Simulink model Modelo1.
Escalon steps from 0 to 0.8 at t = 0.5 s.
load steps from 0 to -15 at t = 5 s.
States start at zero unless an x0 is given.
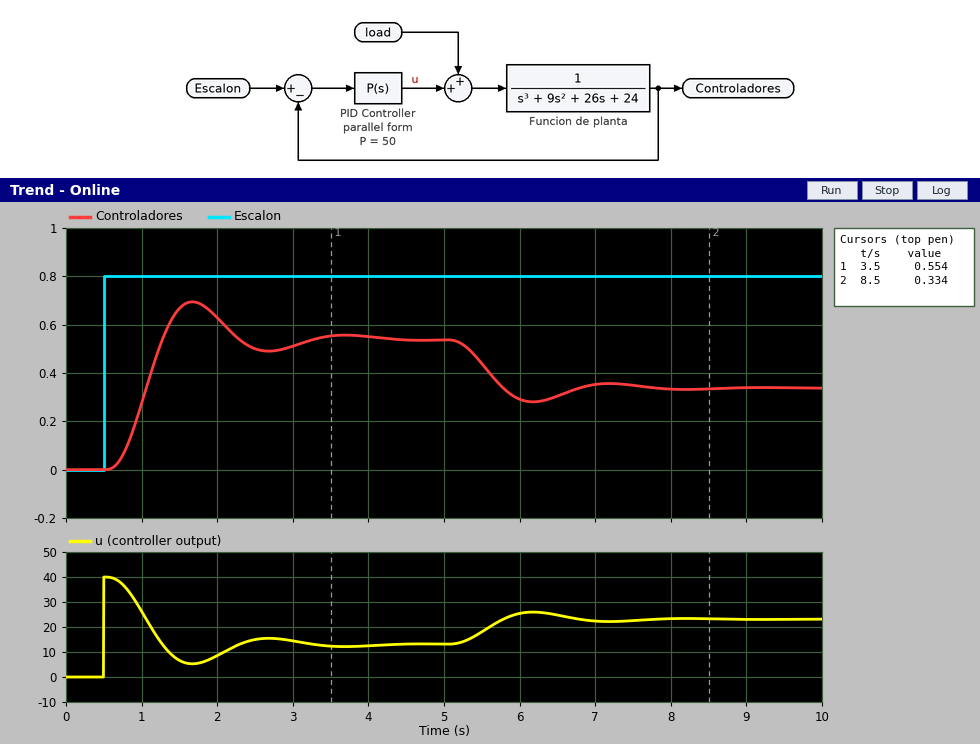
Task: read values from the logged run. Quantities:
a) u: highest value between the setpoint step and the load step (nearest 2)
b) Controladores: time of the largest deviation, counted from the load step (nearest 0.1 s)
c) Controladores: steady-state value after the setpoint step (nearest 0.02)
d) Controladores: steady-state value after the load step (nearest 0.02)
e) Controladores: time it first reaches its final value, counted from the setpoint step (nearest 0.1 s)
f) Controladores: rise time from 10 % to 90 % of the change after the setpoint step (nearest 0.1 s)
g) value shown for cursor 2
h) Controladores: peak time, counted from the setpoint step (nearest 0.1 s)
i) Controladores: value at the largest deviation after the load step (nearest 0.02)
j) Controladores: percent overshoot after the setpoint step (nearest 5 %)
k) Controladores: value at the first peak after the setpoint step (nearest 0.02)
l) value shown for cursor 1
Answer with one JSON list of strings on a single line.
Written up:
["40", "1.2 s", "0.54", "0.34", "0.8 s", "0.5 s", "0.334", "1.2 s", "0.28", "30 %", "0.70", "0.554"]
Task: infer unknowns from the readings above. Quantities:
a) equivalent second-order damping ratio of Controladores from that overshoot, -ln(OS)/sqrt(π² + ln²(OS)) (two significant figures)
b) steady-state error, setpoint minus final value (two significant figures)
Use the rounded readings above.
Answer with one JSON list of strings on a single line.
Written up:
["0.36", "0.26"]
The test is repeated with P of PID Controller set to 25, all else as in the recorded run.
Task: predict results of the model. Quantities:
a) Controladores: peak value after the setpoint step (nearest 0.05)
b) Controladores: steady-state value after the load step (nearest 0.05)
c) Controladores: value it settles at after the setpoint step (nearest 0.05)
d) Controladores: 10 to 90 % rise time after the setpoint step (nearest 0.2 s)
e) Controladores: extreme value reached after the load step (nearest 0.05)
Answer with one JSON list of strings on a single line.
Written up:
["0.45", "0.10", "0.40", "0.6 s", "0.05"]
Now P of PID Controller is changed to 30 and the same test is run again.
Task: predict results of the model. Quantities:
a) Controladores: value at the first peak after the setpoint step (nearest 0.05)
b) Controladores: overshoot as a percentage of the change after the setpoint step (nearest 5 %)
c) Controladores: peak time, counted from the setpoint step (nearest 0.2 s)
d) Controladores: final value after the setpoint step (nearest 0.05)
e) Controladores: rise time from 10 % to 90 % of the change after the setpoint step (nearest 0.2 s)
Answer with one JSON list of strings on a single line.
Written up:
["0.50", "15 %", "1.4 s", "0.45", "0.6 s"]
